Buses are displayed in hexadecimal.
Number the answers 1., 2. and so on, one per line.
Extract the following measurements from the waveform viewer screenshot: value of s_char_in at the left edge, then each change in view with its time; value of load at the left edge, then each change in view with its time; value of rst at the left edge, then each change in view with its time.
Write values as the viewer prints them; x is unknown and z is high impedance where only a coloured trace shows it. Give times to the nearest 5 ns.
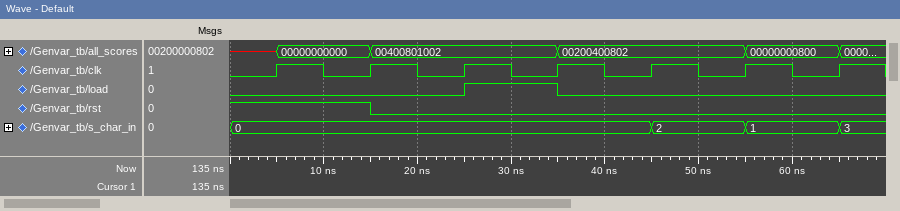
1. 0, 2 at 45 ns, 1 at 55 ns, 3 at 65 ns
2. 0, 1 at 25 ns, 0 at 35 ns
3. 1, 0 at 15 ns
